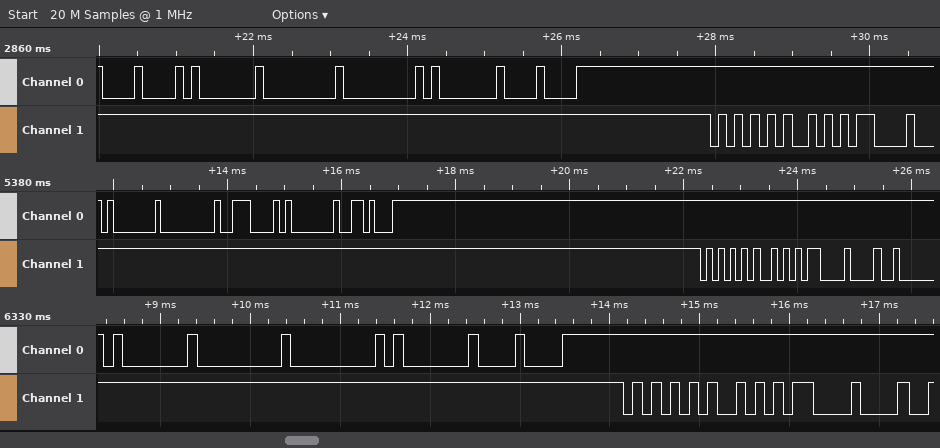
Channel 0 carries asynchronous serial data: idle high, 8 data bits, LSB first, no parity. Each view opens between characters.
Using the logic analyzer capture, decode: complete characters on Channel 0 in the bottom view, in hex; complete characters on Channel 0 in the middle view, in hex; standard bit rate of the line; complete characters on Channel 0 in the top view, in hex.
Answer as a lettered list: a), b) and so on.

a) 01, 00, 00, 01, 08
b) 01, 00, 0E, 01, 16
c) 9600 baud
d) 08, 01, 00, 00, 01, 08
